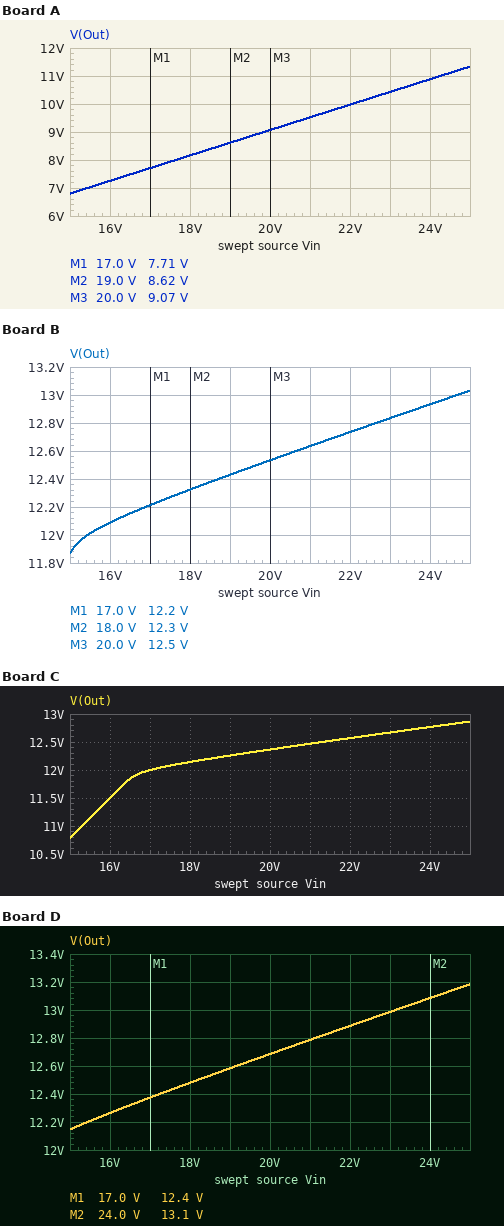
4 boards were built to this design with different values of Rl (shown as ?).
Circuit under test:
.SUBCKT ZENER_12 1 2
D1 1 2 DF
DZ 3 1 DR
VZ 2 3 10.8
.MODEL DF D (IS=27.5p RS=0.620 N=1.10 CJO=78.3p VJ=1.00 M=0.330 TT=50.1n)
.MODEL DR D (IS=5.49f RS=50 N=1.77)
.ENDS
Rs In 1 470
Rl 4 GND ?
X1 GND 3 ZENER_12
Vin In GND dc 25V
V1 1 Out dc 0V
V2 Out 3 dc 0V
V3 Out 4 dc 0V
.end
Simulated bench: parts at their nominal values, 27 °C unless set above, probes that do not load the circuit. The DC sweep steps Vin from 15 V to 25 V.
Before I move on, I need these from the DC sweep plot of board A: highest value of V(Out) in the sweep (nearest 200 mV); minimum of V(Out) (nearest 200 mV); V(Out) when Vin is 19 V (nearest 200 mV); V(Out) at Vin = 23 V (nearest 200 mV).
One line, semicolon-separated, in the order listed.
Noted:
11.4 V; 6.8 V; 8.6 V; 10.4 V
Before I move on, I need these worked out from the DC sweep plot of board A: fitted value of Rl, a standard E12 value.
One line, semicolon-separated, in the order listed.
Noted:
390 Ω
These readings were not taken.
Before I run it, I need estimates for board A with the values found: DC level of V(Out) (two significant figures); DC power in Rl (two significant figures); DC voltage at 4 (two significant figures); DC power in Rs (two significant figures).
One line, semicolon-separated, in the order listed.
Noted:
11 V; 330 mW; 11 V; 400 mW
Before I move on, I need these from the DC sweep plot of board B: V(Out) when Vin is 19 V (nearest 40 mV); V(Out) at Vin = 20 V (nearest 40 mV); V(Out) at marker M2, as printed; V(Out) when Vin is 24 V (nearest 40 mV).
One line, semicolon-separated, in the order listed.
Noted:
12.44 V; 12.52 V; 12.3 V; 12.92 V
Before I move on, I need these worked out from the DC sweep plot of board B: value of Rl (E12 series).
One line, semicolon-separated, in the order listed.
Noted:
1.8 kΩ
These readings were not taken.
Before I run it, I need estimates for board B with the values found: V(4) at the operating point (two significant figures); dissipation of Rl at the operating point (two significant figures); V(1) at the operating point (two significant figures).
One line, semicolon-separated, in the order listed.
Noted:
13 V; 94 mW; 13 V
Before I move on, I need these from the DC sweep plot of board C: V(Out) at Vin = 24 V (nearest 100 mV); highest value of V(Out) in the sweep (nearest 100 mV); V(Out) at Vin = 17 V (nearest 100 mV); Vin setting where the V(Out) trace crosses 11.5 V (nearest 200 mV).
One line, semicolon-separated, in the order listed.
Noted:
12.8 V; 12.9 V; 12.0 V; 16.0 V
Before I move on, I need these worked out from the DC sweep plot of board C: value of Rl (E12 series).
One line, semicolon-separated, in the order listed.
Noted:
1.2 kΩ
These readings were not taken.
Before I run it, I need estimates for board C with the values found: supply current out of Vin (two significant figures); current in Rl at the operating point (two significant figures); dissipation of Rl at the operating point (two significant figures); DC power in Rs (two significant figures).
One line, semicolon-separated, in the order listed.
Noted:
26 mA; 11 mA; 140 mW; 310 mW
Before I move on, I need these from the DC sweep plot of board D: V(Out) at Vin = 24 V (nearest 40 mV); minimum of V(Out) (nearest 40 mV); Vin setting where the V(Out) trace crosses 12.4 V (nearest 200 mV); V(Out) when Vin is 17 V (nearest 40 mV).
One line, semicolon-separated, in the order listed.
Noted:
13.08 V; 12.16 V; 17.2 V; 12.36 V
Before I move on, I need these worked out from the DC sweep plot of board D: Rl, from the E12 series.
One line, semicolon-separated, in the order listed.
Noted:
3.3 kΩ
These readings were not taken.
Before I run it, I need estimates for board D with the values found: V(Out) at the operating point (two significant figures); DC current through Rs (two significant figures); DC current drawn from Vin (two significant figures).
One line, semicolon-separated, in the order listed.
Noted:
13 V; 25 mA; 25 mA
